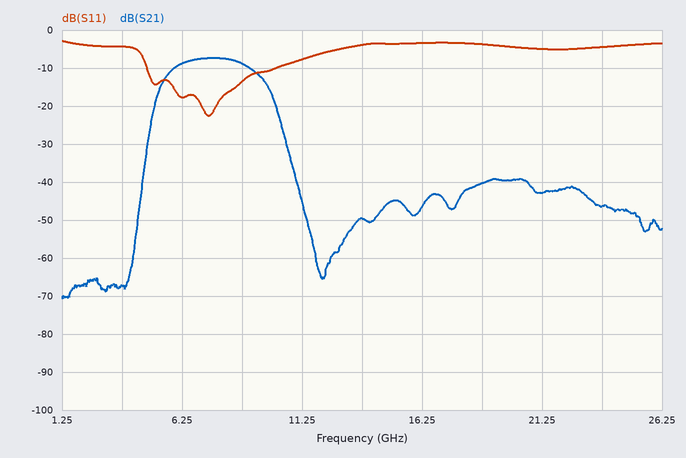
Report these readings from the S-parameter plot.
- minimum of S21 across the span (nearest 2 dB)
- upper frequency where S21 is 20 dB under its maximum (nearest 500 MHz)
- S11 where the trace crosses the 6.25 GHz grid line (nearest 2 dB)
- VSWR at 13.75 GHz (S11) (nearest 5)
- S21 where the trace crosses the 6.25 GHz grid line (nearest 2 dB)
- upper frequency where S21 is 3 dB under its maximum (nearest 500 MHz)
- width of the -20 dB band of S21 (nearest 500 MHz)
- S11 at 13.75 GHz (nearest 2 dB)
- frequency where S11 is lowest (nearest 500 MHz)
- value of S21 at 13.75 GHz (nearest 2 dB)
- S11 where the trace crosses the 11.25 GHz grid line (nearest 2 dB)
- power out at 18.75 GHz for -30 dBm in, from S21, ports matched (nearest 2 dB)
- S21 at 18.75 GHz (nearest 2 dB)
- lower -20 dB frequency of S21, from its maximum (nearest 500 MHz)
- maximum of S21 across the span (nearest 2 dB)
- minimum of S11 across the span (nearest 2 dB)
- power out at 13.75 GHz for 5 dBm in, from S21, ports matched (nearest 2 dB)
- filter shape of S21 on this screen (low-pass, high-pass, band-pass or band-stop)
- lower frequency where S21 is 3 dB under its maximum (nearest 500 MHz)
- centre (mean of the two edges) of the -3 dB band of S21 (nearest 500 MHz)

-70 dB
10.5 GHz
-18 dB
5
-8 dB
9.0 GHz
5.5 GHz
-4 dB
7.5 GHz
-50 dB
-8 dB
-70 dBm
-40 dB
5.0 GHz
-8 dB
-22 dB
-44 dBm
band-pass
6.0 GHz
7.5 GHz
